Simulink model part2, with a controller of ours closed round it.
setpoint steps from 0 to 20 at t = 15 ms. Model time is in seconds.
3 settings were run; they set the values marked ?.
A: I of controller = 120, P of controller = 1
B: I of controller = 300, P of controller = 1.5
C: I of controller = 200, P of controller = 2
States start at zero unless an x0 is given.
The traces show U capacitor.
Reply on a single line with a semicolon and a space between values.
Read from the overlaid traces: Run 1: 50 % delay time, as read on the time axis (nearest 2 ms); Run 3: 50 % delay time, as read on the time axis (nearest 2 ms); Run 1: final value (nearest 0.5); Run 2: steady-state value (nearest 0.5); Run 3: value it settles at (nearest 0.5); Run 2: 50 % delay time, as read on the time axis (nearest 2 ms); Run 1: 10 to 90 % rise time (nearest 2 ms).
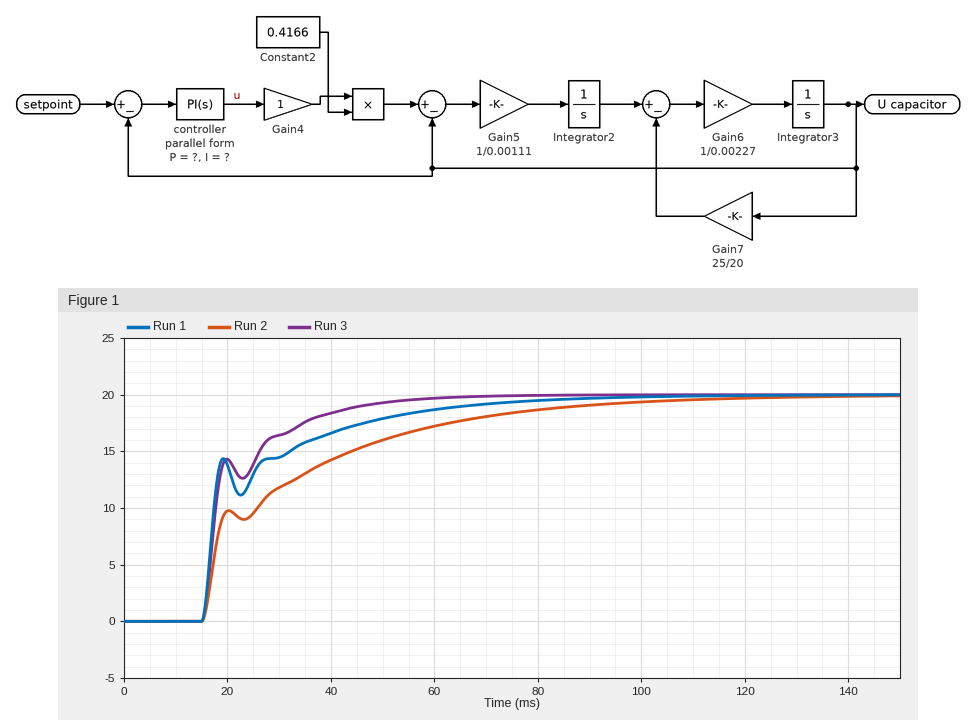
18 ms; 18 ms; 20.0; 20.0; 20.0; 26 ms; 36 ms
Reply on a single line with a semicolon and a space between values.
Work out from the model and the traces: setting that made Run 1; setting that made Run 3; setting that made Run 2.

C; B; A
